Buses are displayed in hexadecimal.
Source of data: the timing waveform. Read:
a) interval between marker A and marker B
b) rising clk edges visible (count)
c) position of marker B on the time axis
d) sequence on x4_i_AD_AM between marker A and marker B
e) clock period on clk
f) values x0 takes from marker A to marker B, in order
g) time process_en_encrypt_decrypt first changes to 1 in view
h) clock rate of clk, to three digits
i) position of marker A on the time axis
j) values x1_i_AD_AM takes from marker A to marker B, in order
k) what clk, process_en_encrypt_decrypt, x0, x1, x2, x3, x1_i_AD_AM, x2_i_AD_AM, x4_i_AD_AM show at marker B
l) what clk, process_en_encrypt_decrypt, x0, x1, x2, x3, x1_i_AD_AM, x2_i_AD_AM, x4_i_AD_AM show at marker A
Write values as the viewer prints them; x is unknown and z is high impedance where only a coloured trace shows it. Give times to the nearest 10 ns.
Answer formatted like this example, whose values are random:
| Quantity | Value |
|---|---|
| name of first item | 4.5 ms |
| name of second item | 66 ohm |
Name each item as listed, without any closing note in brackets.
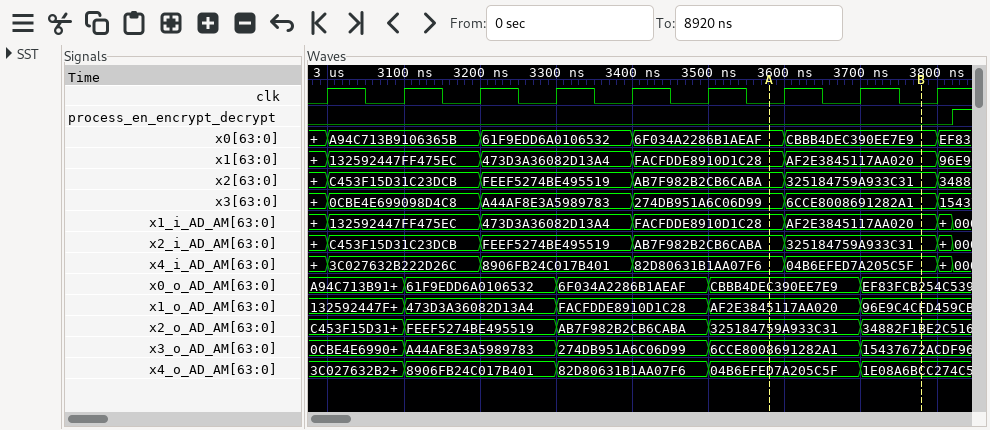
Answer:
| Quantity | Value |
|---|---|
| interval between marker A and marker B | 200 ns |
| rising clk edges visible | 9 |
| position of marker B on the time axis | 3780 ns |
| sequence on x4_i_AD_AM between marker A and marker B | 82D80631B1AA07F6, 04B6EFED7A205C5F |
| clock period on clk | 100 ns |
| values x0 takes from marker A to marker B, in order | 6F034A2286B1AEAF, CBBB4DEC390EE7E9 |
| time process_en_encrypt_decrypt first changes to 1 in view | 3820 ns |
| clock rate of clk, to three digits | 10.0 MHz |
| position of marker A on the time axis | 3580 ns |
| values x1_i_AD_AM takes from marker A to marker B, in order | FACFDDE8910D1C28, AF2E3845117AA020 |
| what clk, process_en_encrypt_decrypt, x0, x1, x2, x3, x1_i_AD_AM, x2_i_AD_AM, x4_i_AD_AM show at marker B | clk=0, process_en_encrypt_decrypt=0, x0=CBBB4DEC390EE7E9, x1=AF2E3845117AA020, x2=325184759A933C31, x3=6CCE8008691282A1, x1_i_AD_AM=AF2E3845117AA020, x2_i_AD_AM=325184759A933C31, x4_i_AD_AM=04B6EFED7A205C5F |
| what clk, process_en_encrypt_decrypt, x0, x1, x2, x3, x1_i_AD_AM, x2_i_AD_AM, x4_i_AD_AM show at marker A | clk=0, process_en_encrypt_decrypt=0, x0=6F034A2286B1AEAF, x1=FACFDDE8910D1C28, x2=AB7F982B2CB6CABA, x3=274DB951A6C06D99, x1_i_AD_AM=FACFDDE8910D1C28, x2_i_AD_AM=AB7F982B2CB6CABA, x4_i_AD_AM=82D80631B1AA07F6 |
